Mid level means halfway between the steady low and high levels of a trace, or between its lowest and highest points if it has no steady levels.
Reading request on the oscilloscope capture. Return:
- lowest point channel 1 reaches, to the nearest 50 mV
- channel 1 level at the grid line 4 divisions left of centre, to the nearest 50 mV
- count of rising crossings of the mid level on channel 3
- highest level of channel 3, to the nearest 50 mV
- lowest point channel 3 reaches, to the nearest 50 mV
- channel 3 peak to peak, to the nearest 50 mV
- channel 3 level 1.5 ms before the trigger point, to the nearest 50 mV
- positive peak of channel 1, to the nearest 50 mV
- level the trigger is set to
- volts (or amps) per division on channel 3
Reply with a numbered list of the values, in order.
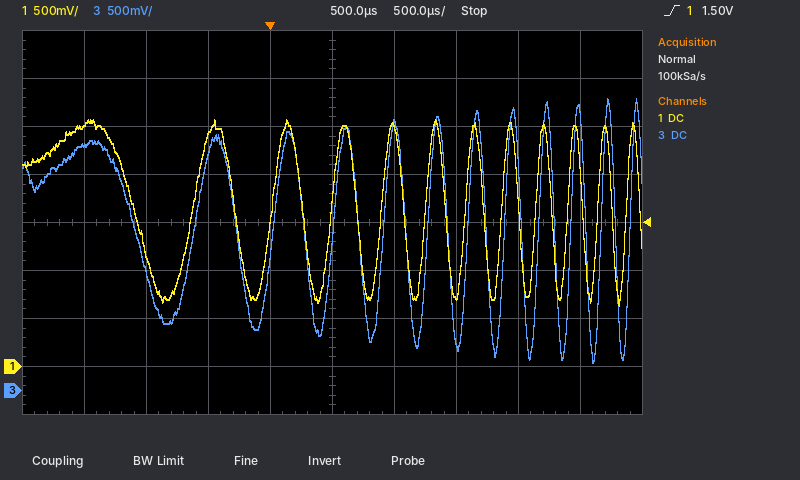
1. 650 mV
2. 2.50 V
3. 11
4. 3.05 V
5. 300 mV
6. 2.75 V
7. 2.55 V
8. 2.55 V
9. 1.50 V
10. 500 mV
